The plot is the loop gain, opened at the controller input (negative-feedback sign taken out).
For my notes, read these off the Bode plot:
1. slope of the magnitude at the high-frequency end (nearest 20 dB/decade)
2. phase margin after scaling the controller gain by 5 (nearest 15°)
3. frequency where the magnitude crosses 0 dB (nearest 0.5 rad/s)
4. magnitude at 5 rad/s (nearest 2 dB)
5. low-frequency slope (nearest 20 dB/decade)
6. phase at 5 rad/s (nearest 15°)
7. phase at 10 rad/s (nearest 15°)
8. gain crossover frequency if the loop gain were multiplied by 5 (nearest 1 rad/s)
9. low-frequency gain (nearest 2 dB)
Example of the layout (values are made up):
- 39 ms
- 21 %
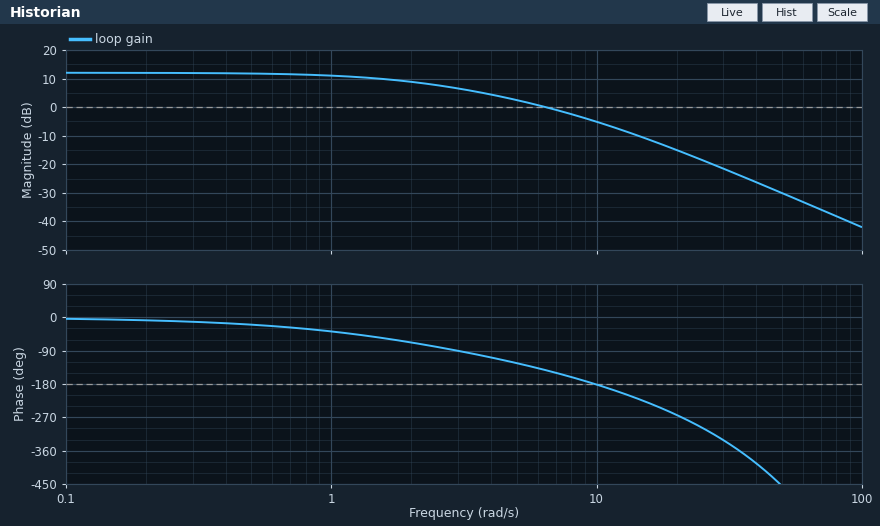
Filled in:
- -40 dB/decade
- -75°
- 6.5 rad/s
- 2 dB
- 0 dB/decade
- -120°
- -180°
- 19 rad/s
- 12 dB
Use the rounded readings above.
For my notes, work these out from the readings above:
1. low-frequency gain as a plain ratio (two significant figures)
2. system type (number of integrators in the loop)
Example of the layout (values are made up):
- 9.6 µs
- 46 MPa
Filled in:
- 4.0
- 0
